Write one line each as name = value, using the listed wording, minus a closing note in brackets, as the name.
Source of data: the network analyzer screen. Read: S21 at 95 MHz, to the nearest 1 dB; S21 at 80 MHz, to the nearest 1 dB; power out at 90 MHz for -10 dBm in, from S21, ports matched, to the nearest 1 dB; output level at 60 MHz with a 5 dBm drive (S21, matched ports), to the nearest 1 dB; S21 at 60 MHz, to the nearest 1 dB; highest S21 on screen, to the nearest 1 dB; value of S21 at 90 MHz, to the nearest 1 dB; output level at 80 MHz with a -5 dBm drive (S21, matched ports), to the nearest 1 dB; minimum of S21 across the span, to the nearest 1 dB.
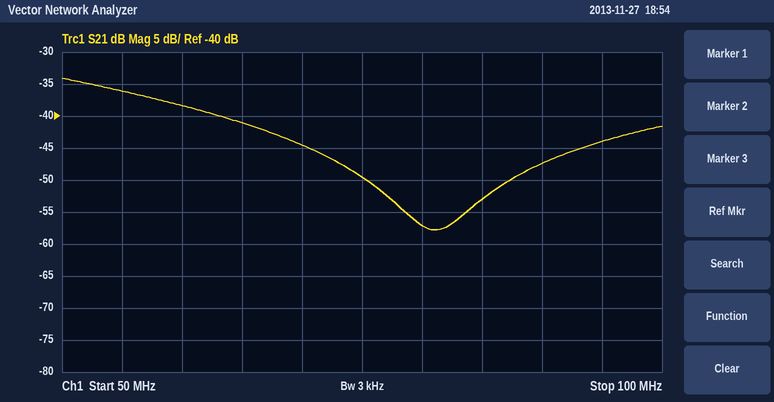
S21 at 95 MHz, to the nearest 1 dB = -44 dB
S21 at 80 MHz, to the nearest 1 dB = -57 dB
power out at 90 MHz for -10 dBm in, from S21, ports matched, to the nearest 1 dB = -57 dBm
output level at 60 MHz with a 5 dBm drive (S21, matched ports), to the nearest 1 dB = -33 dBm
S21 at 60 MHz, to the nearest 1 dB = -38 dB
highest S21 on screen, to the nearest 1 dB = -34 dB
value of S21 at 90 MHz, to the nearest 1 dB = -47 dB
output level at 80 MHz with a -5 dBm drive (S21, matched ports), to the nearest 1 dB = -62 dBm
minimum of S21 across the span, to the nearest 1 dB = -58 dB
